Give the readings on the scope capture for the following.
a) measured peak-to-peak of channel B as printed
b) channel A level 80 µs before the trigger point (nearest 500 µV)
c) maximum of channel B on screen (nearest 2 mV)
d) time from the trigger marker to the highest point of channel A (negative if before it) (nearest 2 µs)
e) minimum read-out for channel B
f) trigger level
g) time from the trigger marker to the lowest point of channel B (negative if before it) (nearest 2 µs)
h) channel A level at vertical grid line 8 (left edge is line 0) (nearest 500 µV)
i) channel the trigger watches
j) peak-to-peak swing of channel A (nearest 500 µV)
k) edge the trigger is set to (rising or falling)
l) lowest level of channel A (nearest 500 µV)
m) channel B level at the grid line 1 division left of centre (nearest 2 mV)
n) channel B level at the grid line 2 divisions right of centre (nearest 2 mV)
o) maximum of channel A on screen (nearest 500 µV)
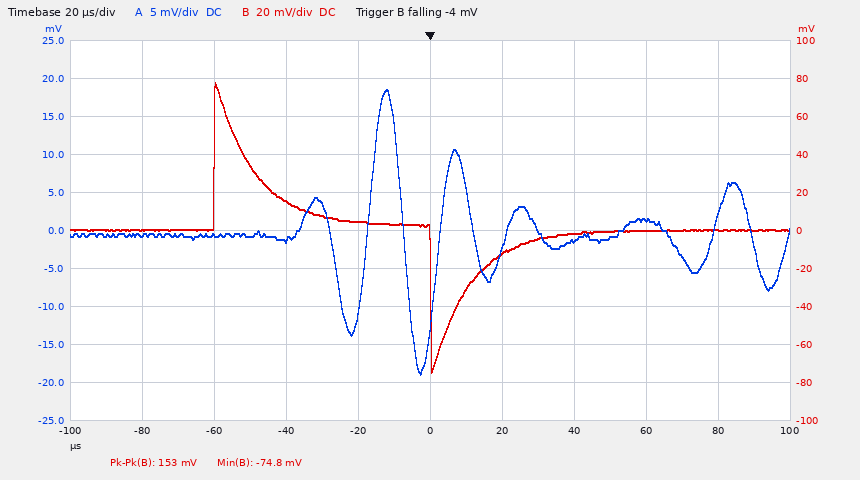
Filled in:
153 mV
-500 µV
78 mV
-12 µs
-74.8 mV
-4 mV
0 µs
1.5 mV
channel B
37.5 mV
falling
-19.0 mV
4 mV
-2 mV
18.5 mV
